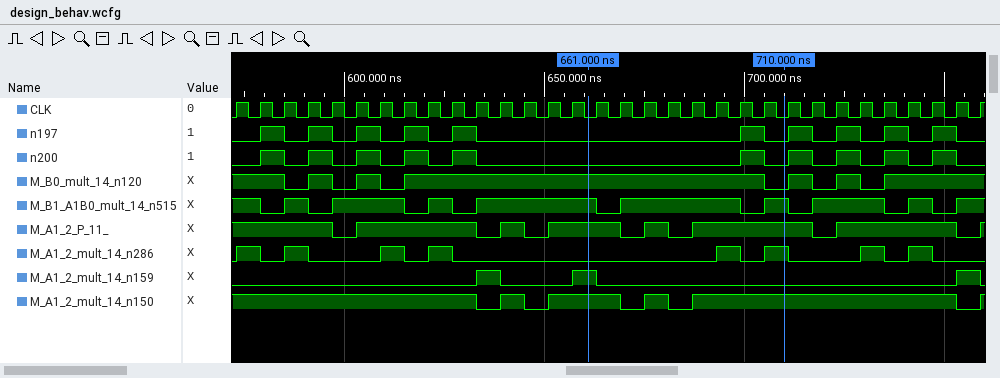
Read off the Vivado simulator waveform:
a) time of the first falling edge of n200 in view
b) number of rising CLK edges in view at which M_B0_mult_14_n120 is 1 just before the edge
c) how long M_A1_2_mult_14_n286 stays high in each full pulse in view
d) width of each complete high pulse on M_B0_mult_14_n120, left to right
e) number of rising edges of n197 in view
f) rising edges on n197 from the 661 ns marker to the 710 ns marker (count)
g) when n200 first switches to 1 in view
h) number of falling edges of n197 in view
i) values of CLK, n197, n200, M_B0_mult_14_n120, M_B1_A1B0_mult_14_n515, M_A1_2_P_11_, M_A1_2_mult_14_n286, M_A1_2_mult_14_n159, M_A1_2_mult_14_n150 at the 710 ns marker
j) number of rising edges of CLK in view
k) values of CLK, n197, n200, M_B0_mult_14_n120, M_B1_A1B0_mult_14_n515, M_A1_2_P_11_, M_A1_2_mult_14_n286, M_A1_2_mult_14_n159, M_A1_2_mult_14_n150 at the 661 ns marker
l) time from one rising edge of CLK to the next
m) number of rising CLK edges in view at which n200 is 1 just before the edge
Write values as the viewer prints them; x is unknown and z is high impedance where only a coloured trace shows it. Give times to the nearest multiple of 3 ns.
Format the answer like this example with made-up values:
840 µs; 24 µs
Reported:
585 ns; 26; 6 ns, 6 ns, 6 ns, 6 ns, 6 ns, 6 ns, 6 ns, 6 ns; 6 ns, 6 ns, 90 ns, 6 ns, 6 ns; 10; 1; 579 ns; 10; CLK=0, n197=0, n200=0, M_B0_mult_14_n120=0, M_B1_A1B0_mult_14_n515=1, M_A1_2_P_11_=1, M_A1_2_mult_14_n286=1, M_A1_2_mult_14_n159=0, M_A1_2_mult_14_n150=1; 32; CLK=0, n197=0, n200=0, M_B0_mult_14_n120=1, M_B1_A1B0_mult_14_n515=1, M_A1_2_P_11_=1, M_A1_2_mult_14_n286=0, M_A1_2_mult_14_n159=1, M_A1_2_mult_14_n150=1; 6 ns; 10
